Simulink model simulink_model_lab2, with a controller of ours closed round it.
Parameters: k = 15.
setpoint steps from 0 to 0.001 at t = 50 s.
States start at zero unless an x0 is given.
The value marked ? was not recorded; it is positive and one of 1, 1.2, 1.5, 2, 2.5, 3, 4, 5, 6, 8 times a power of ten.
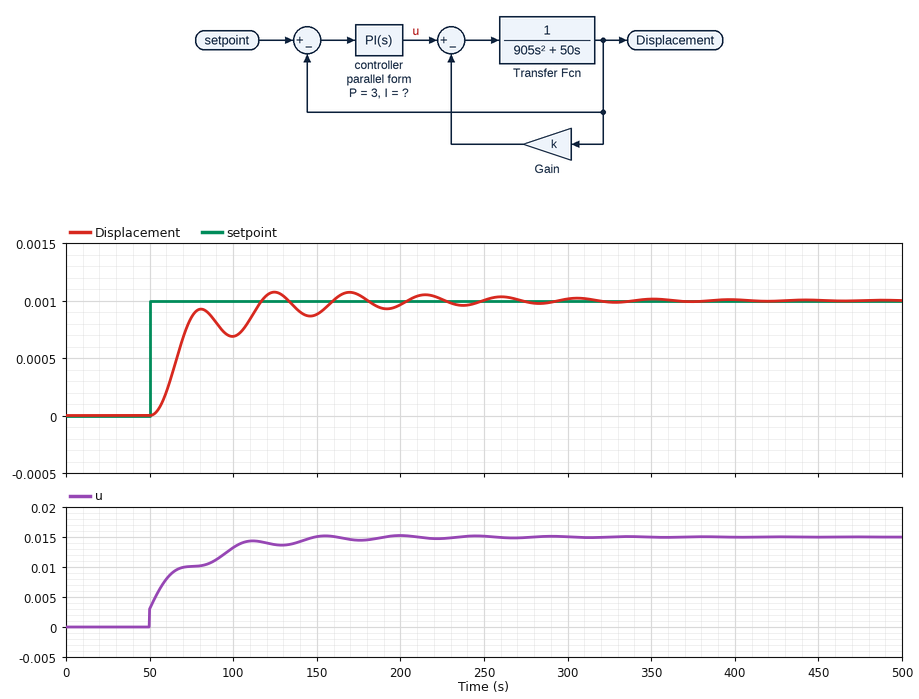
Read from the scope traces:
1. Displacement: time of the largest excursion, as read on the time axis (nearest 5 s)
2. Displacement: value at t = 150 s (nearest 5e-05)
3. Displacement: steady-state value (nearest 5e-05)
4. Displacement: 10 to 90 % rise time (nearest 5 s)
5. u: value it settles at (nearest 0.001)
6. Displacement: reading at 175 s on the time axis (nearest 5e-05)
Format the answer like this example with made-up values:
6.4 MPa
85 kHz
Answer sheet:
125 s
0.00090
0.00100
20 s
0.015
0.00105
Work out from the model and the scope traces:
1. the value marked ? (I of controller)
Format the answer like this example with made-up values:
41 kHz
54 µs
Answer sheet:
0.6
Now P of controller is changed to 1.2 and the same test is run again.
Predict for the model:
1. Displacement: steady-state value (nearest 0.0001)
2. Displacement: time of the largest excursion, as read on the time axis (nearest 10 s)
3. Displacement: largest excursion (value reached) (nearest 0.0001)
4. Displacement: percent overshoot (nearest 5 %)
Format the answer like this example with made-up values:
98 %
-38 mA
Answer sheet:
0.0010
130 s
0.0011
10 %
